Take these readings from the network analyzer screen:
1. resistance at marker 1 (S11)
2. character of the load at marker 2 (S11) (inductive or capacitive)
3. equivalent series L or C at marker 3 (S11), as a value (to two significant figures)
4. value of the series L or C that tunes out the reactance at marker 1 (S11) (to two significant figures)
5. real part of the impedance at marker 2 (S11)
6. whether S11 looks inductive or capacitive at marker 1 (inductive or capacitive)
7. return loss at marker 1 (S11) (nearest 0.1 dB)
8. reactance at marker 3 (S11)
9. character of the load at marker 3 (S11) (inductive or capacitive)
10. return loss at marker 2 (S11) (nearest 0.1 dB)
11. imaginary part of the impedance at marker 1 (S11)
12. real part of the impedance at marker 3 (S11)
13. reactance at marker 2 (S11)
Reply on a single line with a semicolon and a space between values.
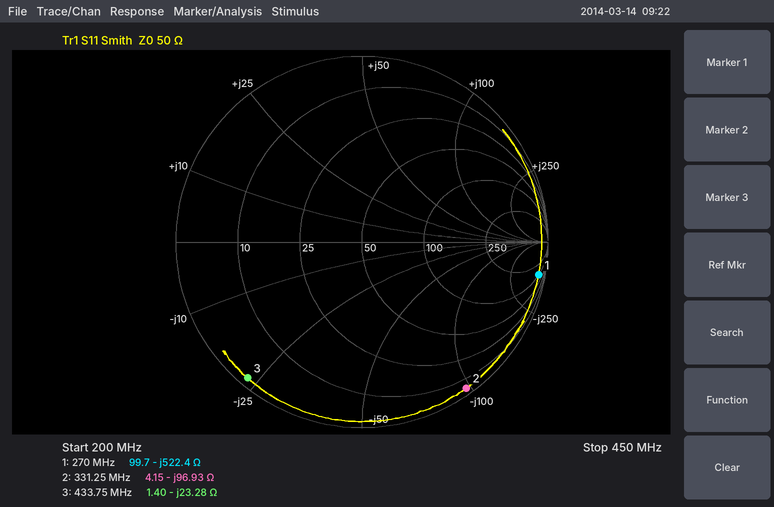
99.7 Ω; capacitive; 16 pF; 310 nH; 4.15 Ω; capacitive; 0.3 dB; -23.28 Ω; capacitive; 0.3 dB; -522.4 Ω; 1.40 Ω; -96.93 Ω
